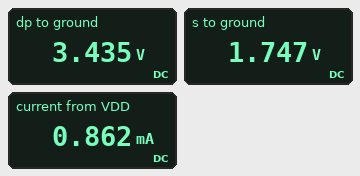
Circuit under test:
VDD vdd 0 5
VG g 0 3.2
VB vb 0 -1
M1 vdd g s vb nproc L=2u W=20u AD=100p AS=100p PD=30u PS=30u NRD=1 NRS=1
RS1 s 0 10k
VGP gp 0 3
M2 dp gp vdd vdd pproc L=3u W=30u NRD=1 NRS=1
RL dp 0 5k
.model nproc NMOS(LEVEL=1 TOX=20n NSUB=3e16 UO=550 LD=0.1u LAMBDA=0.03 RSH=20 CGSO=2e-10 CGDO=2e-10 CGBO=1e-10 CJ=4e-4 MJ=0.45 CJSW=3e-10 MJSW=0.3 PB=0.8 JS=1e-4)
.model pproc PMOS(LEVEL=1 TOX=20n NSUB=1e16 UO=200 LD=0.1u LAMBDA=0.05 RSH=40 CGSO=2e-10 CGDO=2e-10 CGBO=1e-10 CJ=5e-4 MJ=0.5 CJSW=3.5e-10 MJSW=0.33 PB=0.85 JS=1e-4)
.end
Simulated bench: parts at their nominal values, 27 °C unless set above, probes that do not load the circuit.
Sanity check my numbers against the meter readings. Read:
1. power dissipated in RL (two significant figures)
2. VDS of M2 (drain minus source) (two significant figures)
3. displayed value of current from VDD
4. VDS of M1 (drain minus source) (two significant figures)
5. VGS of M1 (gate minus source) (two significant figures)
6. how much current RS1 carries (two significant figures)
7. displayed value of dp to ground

2.4 mW
-1.6 V
0.862 mA
3.3 V
1.5 V
170 µA
3.435 V
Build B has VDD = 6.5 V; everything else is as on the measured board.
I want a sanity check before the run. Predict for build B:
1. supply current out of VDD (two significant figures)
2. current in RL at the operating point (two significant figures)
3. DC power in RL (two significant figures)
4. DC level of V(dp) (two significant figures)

1.3 mA
1.1 mA
5.9 mW
5.4 V
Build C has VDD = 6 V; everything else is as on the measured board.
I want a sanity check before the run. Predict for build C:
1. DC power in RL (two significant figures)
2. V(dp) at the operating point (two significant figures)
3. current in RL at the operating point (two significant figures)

4.7 mW
4.9 V
970 µA
